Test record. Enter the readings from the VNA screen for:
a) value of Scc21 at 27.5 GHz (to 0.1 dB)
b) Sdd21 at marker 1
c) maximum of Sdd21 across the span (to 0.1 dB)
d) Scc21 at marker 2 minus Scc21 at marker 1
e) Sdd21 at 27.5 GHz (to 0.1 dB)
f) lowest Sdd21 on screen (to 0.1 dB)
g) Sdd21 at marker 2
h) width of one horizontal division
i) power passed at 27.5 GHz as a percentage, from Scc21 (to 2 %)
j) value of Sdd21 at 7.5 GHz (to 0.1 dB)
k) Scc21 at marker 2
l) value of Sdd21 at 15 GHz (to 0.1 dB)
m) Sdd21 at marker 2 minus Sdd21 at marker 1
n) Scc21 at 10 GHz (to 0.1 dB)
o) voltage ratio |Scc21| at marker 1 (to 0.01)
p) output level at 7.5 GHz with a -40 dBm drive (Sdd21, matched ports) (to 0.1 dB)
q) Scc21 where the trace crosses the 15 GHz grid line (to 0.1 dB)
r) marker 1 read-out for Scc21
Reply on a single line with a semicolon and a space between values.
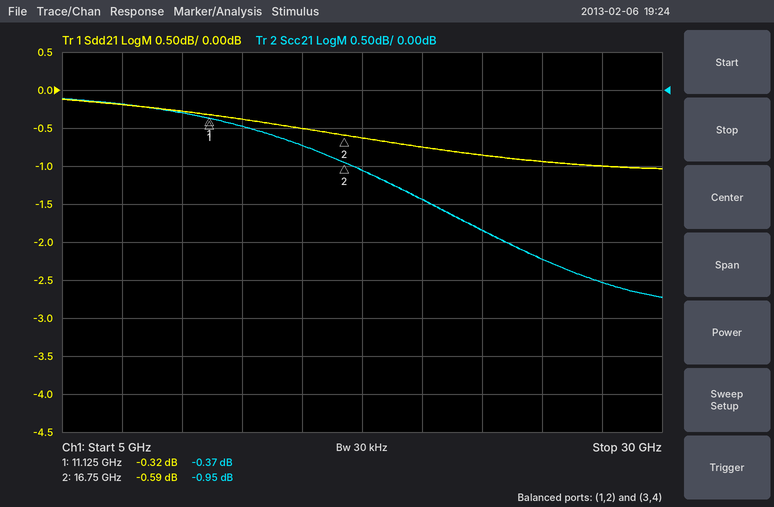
-2.5 dB; -0.32 dB; -0.1 dB; -0.58 dB; -1.0 dB; -1.0 dB; -0.59 dB; 2.5 GHz; 56 %; -0.2 dB; -0.95 dB; -0.5 dB; -0.27 dB; -0.3 dB; 0.96; -40.2 dBm; -0.7 dB; -0.37 dB
